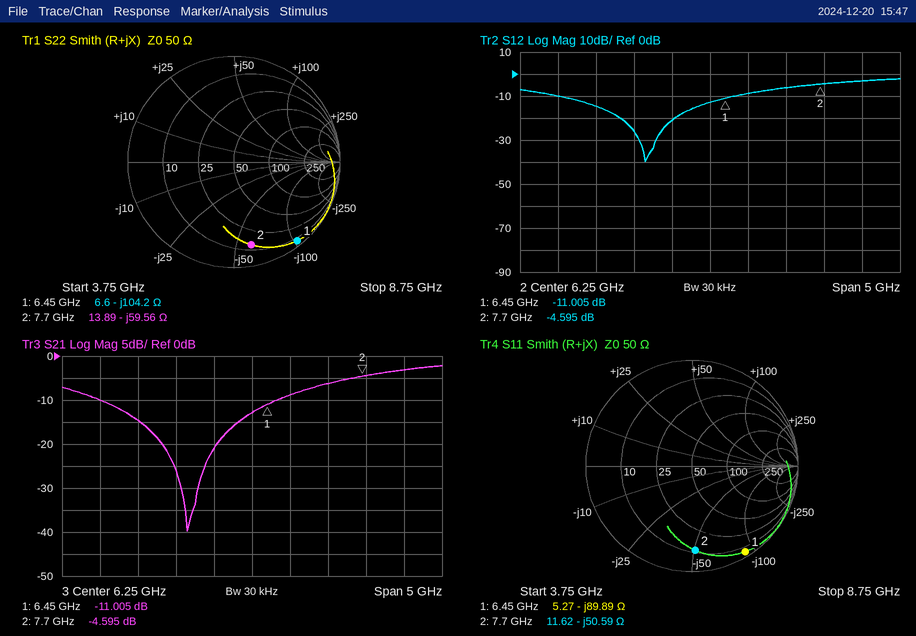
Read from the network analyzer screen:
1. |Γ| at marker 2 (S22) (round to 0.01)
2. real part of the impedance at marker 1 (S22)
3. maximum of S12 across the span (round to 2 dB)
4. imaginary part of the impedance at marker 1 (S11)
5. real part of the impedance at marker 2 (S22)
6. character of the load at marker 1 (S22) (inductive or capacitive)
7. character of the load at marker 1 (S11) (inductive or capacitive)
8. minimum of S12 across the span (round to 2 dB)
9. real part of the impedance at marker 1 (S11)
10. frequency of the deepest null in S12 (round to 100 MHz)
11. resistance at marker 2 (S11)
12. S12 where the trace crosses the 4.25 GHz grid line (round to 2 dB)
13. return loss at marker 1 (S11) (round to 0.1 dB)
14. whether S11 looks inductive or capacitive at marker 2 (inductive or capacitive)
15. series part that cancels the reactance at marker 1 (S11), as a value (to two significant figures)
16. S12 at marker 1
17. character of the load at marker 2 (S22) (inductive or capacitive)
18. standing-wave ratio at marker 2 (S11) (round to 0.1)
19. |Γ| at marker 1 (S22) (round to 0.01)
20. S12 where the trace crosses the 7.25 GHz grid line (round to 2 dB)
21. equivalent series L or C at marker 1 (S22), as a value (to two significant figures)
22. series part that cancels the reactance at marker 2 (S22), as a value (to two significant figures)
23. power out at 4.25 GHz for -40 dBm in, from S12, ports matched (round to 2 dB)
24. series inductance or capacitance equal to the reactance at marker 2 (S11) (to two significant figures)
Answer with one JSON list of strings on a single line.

["0.80", "6.6 Ω", "-2 dB", "-89.89 Ω", "13.89 Ω", "capacitive", "capacitive", "-40 dB", "5.27 Ω", "5.4 GHz", "11.62 Ω", "-10 dB", "0.4 dB", "capacitive", "2.2 nH", "-11.005 dB", "capacitive", "8.8", "0.95", "-6 dB", "240 fF", "1.2 nH", "-50 dBm", "410 fF"]
